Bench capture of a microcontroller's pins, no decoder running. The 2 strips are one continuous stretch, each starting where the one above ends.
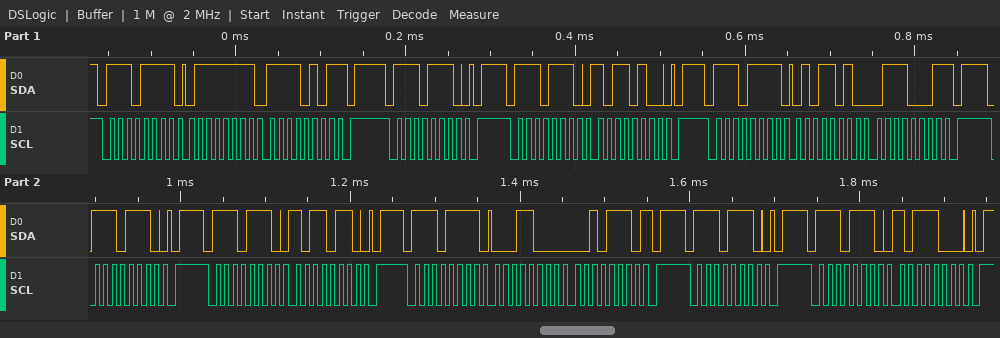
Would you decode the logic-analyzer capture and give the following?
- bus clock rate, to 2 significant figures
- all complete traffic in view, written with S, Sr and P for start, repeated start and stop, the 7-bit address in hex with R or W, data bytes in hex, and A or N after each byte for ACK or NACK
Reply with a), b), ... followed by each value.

a) 100 kHz
b) S 77R A 7F A F5 N P S 77W A P S 77W A B4 A P S 77R A 5A A 71 N P S 77W A P S 77W A B6 A P S 77R A 18 A 2E N P S 77W A P S 77W A B8 A P
